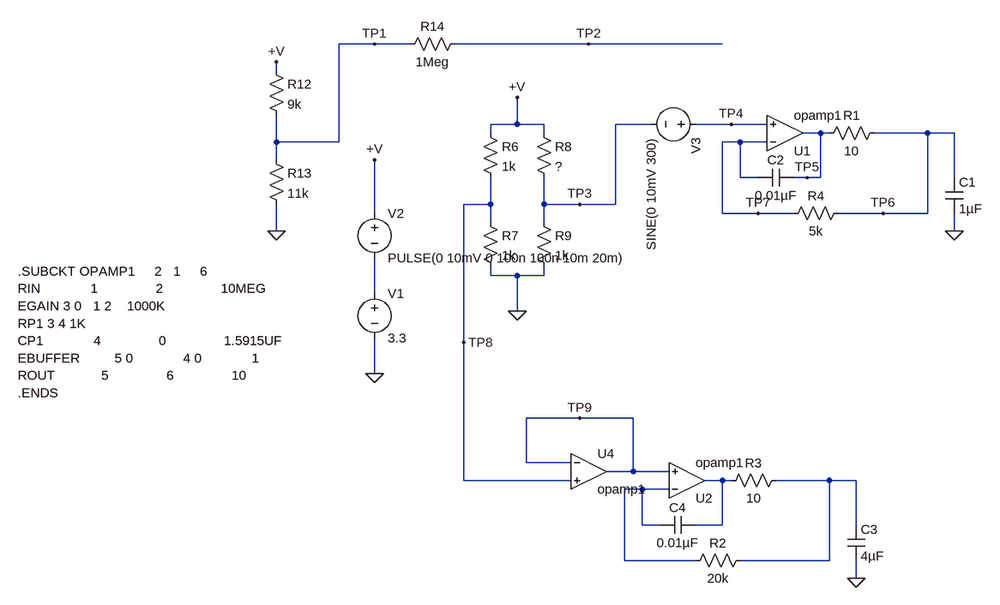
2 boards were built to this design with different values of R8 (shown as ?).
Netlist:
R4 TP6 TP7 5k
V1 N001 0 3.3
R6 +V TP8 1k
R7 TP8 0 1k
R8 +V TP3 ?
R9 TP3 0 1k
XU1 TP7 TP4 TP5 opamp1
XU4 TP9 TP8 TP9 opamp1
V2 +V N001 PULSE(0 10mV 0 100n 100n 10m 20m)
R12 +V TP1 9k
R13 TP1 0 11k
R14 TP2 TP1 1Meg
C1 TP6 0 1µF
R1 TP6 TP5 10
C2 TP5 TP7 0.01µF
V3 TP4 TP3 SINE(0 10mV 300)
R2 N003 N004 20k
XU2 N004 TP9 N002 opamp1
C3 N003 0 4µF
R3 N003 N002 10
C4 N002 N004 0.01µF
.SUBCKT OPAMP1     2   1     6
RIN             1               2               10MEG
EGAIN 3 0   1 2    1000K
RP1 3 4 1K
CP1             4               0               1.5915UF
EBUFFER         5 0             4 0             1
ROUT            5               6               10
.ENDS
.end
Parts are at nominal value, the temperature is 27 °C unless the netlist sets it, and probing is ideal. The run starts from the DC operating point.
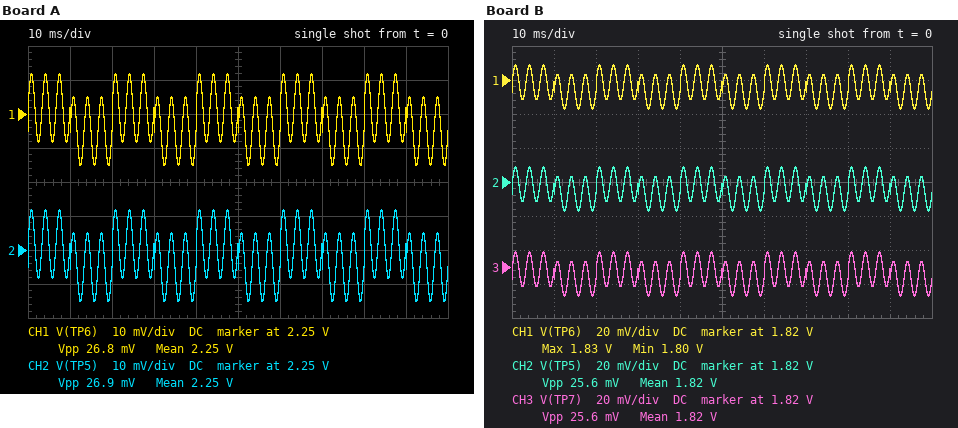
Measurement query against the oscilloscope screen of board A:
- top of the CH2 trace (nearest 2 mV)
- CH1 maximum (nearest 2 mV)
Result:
2.262 V
2.262 V
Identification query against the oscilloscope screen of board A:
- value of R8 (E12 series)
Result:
470 Ω
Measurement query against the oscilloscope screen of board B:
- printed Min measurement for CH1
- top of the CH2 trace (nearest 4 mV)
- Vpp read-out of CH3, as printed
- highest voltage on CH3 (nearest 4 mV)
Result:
1.80 V
1.828 V
25.6 mV
1.828 V
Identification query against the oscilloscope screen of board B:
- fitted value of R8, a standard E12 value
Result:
820 Ω
